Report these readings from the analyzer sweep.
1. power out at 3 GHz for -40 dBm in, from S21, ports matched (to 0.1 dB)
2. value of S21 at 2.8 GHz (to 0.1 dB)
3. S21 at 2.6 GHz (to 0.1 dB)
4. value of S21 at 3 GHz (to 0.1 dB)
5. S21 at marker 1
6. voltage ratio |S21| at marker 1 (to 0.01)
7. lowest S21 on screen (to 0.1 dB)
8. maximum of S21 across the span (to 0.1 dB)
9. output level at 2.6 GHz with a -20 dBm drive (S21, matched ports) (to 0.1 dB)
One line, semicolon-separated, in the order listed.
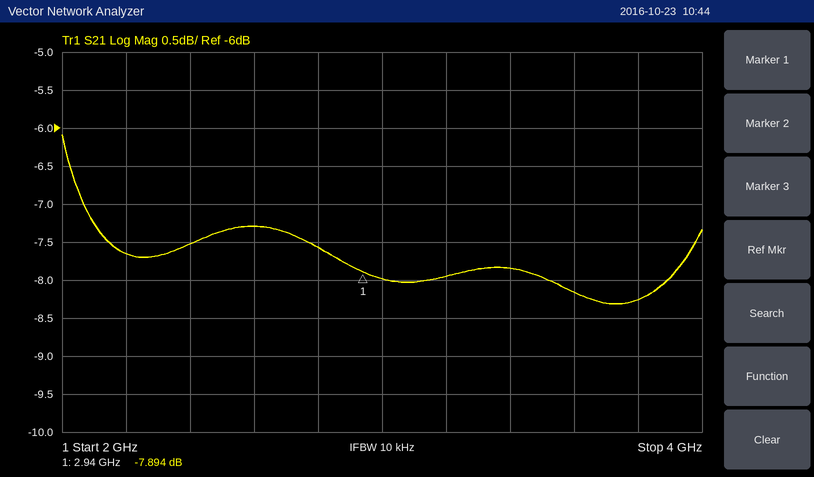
-48.0 dBm; -7.6 dB; -7.3 dB; -8.0 dB; -7.894 dB; 0.40; -8.3 dB; -6.1 dB; -27.3 dBm
